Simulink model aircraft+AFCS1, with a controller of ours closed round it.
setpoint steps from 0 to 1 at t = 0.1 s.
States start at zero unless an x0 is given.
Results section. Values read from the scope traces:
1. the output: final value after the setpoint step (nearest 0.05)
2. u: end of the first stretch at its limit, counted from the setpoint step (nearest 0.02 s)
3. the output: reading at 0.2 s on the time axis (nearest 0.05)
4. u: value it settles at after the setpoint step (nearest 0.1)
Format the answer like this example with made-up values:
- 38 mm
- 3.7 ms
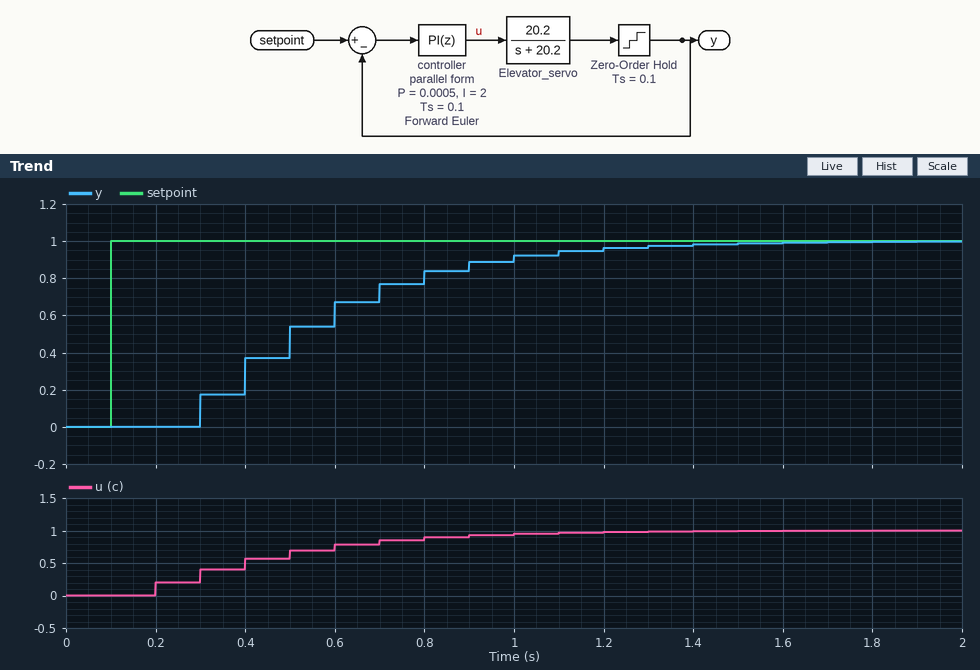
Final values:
- 1.00
- 0.10 s
- 0.00
- 1.0
